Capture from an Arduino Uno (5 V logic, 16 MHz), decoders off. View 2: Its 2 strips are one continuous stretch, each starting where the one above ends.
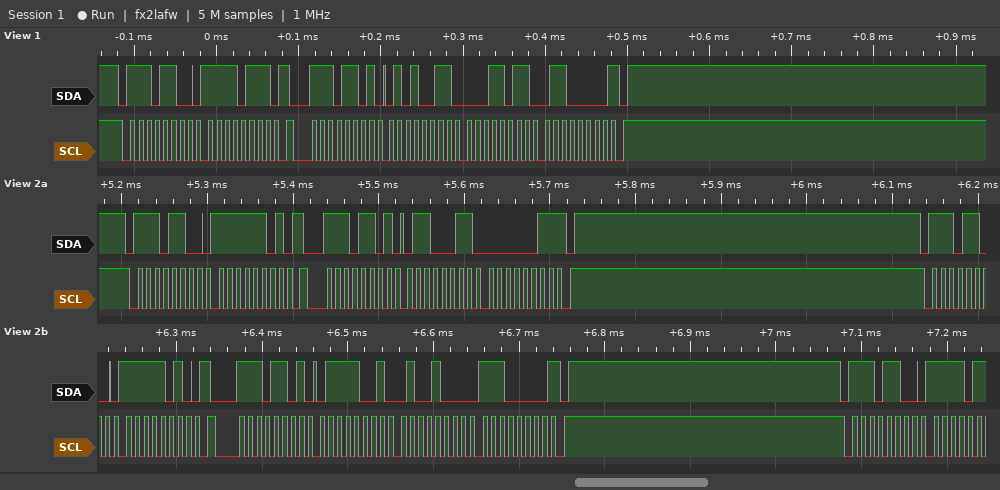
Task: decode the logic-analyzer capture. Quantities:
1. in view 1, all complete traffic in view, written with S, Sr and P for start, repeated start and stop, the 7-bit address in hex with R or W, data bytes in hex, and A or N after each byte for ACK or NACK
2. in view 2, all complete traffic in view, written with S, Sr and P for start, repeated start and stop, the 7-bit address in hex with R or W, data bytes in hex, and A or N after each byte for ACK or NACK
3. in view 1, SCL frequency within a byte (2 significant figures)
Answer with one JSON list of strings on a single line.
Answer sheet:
["S 76W A F7 A Sr 76R A 53 A 1B A 60 N P", "S 76W A FD A Sr 76R A 63 A 03 N P S 76W A FA A Sr 76R A 79 A 48 A E0 N P S 76W A", "100 kHz"]
